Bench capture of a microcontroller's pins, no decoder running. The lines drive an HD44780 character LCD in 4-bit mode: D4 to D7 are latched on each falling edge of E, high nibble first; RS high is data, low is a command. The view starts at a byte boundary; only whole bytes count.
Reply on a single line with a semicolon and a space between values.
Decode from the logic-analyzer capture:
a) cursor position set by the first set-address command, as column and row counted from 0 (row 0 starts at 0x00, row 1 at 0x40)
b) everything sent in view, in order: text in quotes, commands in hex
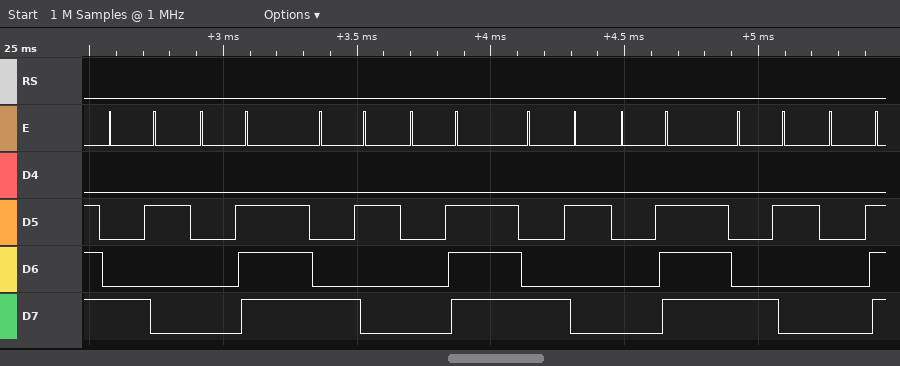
column 2, row 0; 0x82 0x0E 0x82 0x0E 0x82 0x0E 0x82 0x0E
